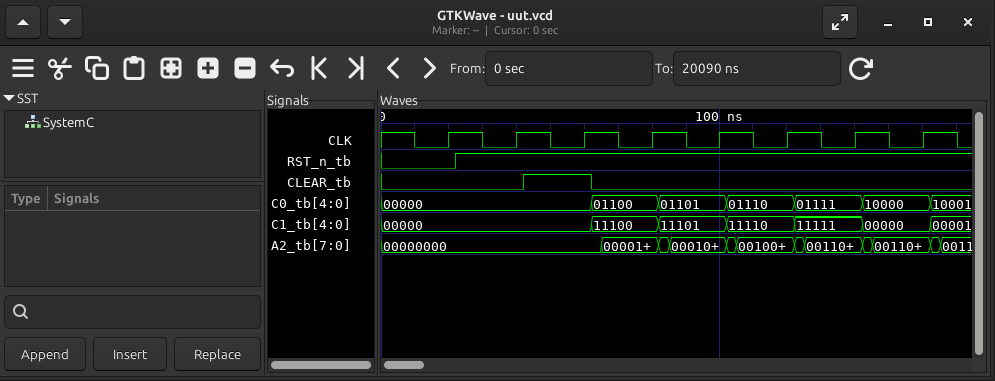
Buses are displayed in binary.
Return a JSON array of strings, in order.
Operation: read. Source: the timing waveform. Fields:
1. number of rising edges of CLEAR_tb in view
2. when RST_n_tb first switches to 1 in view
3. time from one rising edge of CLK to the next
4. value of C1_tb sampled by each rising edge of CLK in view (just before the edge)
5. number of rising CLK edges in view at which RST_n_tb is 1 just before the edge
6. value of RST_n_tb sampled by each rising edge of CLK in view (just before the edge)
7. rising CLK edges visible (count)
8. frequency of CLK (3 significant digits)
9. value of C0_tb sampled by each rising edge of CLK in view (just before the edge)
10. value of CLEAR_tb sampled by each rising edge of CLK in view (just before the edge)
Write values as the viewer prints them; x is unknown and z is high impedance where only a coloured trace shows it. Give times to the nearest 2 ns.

["1", "22 ns", "20 ns", "00000, 00000, 00000, 11100, 11101, 11110, 11111, 00000", "7", "0 1 1 1 1 1 1 1", "8", "50.0 MHz", "00000, 00000, 00000, 01100, 01101, 01110, 01111, 10000", "0 0 1 0 0 0 0 0"]
